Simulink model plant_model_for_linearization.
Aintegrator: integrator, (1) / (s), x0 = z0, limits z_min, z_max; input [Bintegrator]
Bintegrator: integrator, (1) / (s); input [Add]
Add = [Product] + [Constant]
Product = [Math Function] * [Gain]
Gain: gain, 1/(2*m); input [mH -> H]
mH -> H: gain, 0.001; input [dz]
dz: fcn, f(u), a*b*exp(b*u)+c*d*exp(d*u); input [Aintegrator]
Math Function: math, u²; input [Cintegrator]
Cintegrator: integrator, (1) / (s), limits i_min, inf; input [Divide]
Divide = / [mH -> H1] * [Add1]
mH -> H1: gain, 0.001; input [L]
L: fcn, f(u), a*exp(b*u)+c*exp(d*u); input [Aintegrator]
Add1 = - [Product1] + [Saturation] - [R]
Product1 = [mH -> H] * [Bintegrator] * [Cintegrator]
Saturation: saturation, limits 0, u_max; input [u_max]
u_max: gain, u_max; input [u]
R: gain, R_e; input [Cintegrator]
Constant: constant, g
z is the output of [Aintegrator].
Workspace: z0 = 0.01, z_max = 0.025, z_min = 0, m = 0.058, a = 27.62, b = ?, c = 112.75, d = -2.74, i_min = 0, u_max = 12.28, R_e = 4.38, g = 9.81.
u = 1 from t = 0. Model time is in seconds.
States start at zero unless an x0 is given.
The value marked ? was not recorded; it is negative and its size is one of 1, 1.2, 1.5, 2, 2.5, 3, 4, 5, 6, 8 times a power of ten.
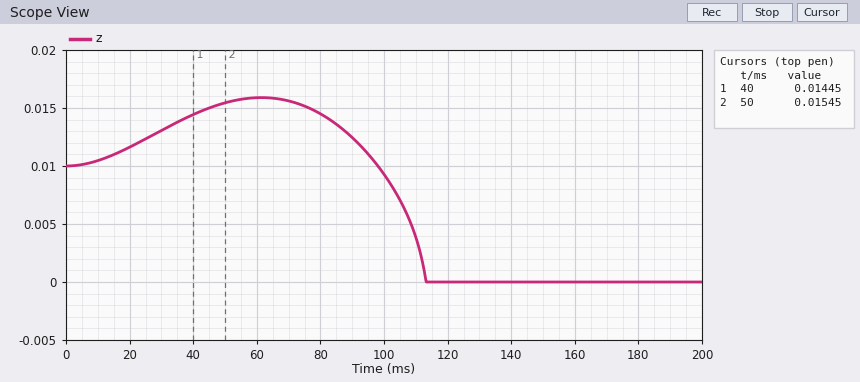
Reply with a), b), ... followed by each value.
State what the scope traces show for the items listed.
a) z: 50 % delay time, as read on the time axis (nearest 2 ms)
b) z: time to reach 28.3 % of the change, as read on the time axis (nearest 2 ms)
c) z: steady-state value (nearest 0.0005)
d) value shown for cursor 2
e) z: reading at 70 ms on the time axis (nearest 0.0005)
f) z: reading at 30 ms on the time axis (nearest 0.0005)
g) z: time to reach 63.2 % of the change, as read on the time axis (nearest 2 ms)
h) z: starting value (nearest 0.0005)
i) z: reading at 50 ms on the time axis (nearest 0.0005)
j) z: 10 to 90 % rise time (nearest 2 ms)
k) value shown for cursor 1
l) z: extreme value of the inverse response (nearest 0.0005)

a) 108 ms
b) 104 ms
c) 0.0000
d) 0.01545
e) 0.0155
f) 0.0130
g) 110 ms
h) 0.0100
i) 0.0155
j) 12 ms
k) 0.01445
l) 0.0160
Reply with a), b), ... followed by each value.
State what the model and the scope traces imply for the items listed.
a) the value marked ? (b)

a) -500
